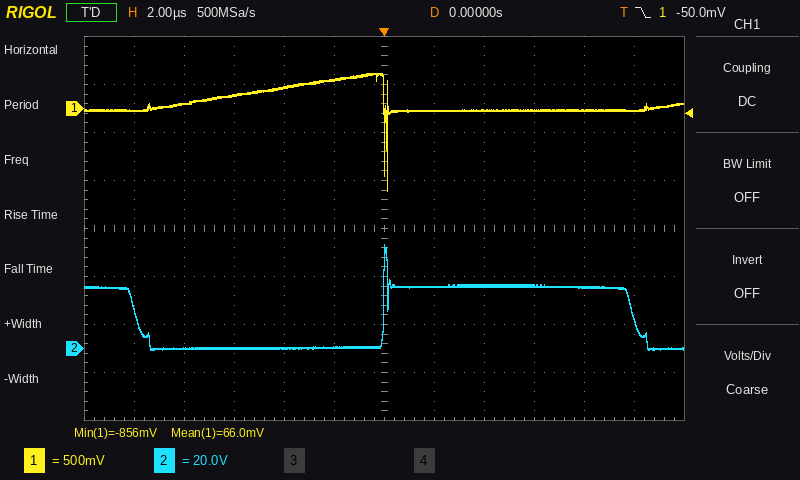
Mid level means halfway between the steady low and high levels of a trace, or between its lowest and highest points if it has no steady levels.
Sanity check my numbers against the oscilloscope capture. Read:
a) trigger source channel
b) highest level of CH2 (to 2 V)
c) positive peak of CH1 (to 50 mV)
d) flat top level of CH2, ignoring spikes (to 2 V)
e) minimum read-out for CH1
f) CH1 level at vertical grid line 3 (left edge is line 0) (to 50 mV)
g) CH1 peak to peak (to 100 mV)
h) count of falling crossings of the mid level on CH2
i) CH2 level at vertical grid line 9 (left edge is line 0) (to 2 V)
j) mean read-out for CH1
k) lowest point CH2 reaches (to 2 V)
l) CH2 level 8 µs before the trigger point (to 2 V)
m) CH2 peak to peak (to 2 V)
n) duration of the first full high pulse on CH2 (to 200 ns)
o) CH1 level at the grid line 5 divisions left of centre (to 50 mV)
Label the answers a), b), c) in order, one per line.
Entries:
a) CH1
b) 44 V
c) 350 mV
d) 26 V
e) -856 mV
f) 150 mV
g) 1.20 V
h) 2
i) 26 V
j) 66.0 mV
k) 0 V
l) 0 V
m) 44 V
n) 10.0 µs
o) 0 mV
